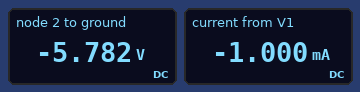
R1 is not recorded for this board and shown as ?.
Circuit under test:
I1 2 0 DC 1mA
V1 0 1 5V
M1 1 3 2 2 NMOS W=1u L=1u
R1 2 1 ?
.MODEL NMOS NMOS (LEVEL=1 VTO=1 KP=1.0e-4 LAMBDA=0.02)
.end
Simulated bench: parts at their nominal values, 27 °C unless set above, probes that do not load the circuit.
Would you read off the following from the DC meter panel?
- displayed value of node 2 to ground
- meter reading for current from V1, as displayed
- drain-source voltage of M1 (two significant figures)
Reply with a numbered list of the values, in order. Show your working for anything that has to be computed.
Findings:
1. -5.782 V
2. -1.000 mA
3. -5 V - (-5.782 V) = 780 mV
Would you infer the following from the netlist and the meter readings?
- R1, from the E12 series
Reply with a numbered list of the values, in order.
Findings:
1. 1.2 kΩ
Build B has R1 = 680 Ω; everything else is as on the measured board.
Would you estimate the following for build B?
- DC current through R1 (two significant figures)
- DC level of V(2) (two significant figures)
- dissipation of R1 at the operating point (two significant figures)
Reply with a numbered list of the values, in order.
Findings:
1. 770 µA
2. -5.5 V
3. 410 µW
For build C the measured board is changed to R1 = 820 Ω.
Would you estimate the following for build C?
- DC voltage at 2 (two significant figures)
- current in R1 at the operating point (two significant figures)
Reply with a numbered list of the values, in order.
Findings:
1. -5.6 V
2. 740 µA
